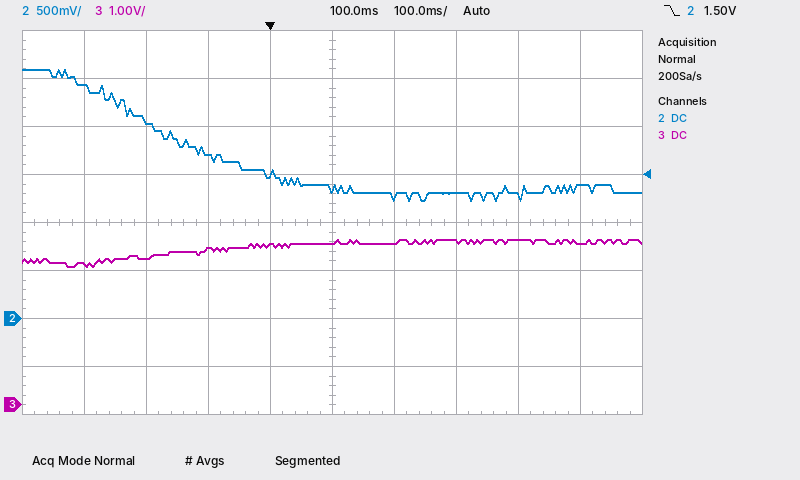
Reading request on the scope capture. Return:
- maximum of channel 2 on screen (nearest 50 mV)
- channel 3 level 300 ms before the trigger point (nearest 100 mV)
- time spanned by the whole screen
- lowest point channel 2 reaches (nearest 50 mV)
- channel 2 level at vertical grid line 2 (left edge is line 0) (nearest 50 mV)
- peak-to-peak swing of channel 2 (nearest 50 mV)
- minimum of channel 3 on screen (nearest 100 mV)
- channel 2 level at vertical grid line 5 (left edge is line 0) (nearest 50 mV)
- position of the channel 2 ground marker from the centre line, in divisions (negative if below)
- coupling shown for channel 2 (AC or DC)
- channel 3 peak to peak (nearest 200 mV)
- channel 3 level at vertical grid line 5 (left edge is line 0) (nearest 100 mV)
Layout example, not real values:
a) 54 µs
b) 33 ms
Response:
a) 2.60 V
b) 2.9 V
c) 1 s
d) 1.25 V
e) 2.05 V
f) 1.35 V
g) 2.9 V
h) 1.35 V
i) -2.0 div
j) DC
k) 600 mV
l) 3.4 V
